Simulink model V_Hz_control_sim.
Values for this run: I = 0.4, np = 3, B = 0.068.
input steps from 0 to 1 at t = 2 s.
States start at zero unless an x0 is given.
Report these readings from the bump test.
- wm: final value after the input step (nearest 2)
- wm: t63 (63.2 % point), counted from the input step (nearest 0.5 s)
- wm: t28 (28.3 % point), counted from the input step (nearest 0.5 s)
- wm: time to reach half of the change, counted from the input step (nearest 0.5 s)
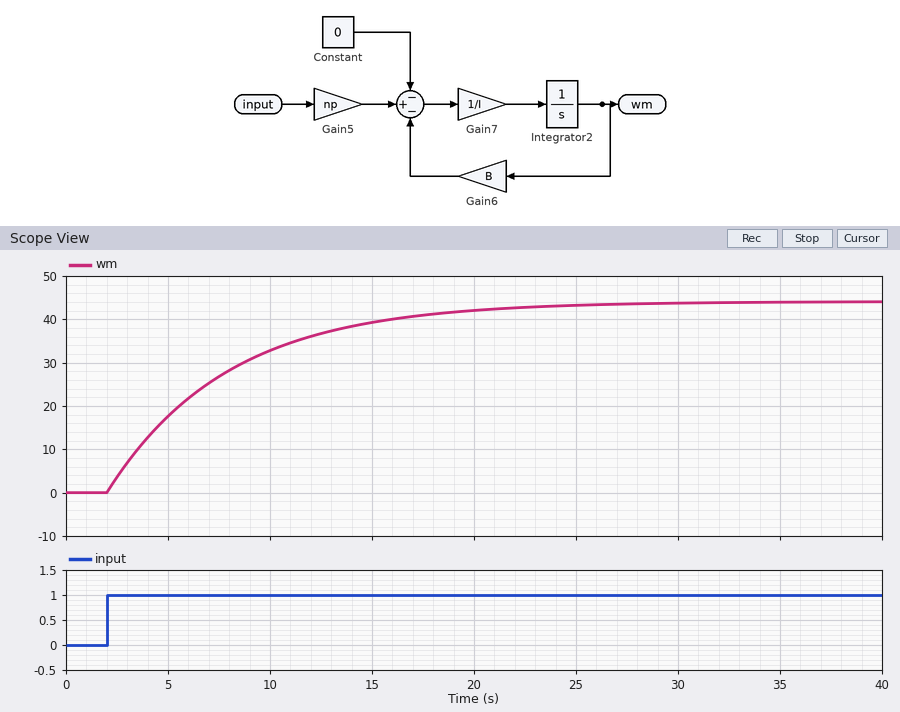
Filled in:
44
6.0 s
2.0 s
4.0 s
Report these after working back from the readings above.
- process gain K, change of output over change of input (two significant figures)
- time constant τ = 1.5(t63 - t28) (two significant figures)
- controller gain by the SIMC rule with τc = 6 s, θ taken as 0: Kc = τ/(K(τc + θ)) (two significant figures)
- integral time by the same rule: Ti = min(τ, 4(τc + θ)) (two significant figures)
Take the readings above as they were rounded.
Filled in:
44
6.0 s
0.023
6.0 s
